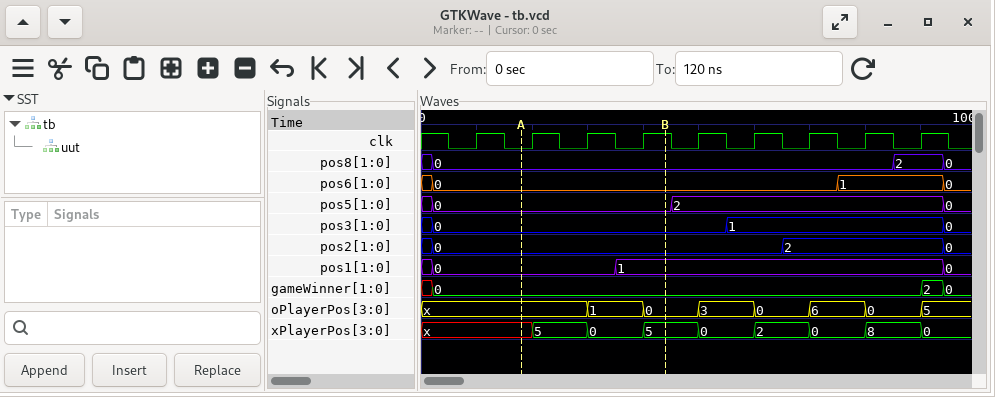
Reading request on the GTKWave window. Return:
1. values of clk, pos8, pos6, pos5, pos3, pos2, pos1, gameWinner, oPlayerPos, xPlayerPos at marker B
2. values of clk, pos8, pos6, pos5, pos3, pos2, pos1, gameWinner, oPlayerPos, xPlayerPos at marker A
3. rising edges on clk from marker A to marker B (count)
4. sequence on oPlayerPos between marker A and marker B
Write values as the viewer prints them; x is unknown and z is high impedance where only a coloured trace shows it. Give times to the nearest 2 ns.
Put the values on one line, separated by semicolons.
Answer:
clk=1, pos8=0, pos6=0, pos5=0, pos3=0, pos2=0, pos1=1, gameWinner=0, oPlayerPos=0, xPlayerPos=5; clk=0, pos8=0, pos6=0, pos5=0, pos3=0, pos2=0, pos1=0, gameWinner=0, oPlayerPos=x, xPlayerPos=x; 3; x, 1, 0
